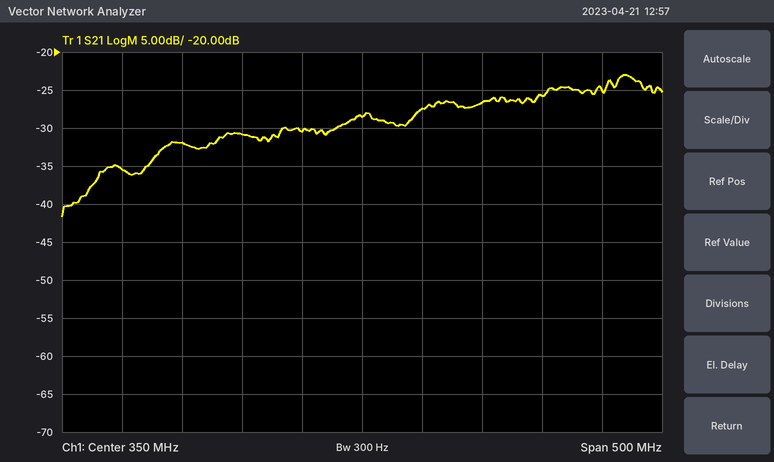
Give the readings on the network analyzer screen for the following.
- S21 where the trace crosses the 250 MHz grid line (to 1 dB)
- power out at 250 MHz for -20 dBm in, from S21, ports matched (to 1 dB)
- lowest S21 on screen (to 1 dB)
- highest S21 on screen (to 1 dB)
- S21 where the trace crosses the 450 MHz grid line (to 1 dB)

-31 dB
-51 dBm
-42 dB
-23 dB
-27 dB
